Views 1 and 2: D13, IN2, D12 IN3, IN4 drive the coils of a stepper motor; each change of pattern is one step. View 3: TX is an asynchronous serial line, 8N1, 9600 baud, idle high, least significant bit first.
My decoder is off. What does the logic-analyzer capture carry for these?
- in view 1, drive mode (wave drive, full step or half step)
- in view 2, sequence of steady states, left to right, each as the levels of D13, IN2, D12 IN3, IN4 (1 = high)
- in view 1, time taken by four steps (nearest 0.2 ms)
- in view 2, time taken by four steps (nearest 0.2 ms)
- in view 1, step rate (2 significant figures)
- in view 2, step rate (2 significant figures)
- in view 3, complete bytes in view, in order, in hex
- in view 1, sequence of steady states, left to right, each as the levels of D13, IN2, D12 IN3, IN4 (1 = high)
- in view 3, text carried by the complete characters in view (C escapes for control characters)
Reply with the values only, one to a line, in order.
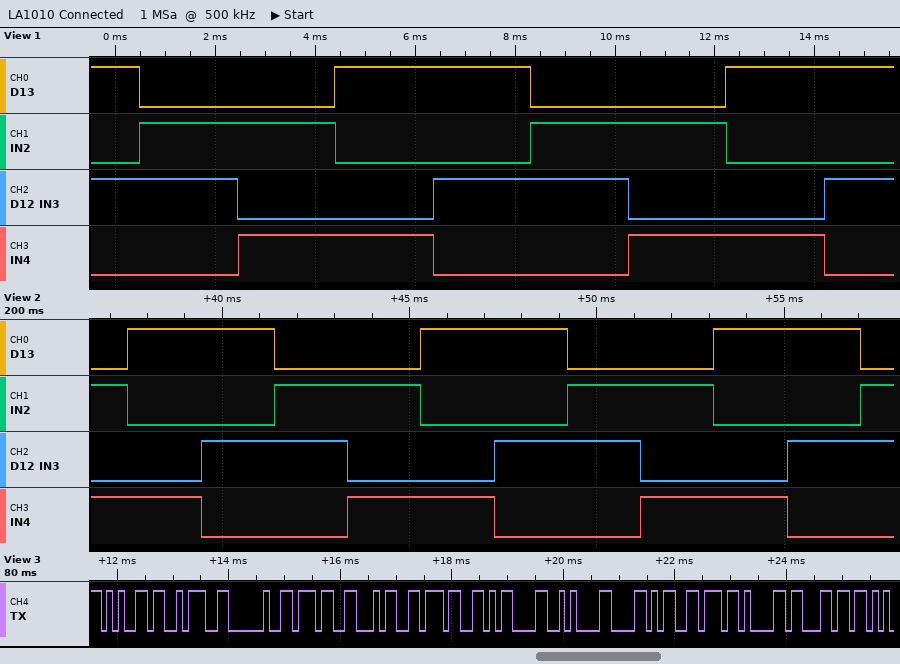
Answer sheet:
full step
0101 1001 1010 0110 0101 1001 1010 0110 0101 1001 1010 0110
7.8 ms
7.8 ms
510 steps/s
510 steps/s
0x65 0x3A 0x20 0x37 0x34 0x37 0x0D 0x0A 0x58 0x76 0x61 0x6C
1010 0110 0101 1001 1010 0110 0101 1001 1010
"e: 747\r\nXval"
